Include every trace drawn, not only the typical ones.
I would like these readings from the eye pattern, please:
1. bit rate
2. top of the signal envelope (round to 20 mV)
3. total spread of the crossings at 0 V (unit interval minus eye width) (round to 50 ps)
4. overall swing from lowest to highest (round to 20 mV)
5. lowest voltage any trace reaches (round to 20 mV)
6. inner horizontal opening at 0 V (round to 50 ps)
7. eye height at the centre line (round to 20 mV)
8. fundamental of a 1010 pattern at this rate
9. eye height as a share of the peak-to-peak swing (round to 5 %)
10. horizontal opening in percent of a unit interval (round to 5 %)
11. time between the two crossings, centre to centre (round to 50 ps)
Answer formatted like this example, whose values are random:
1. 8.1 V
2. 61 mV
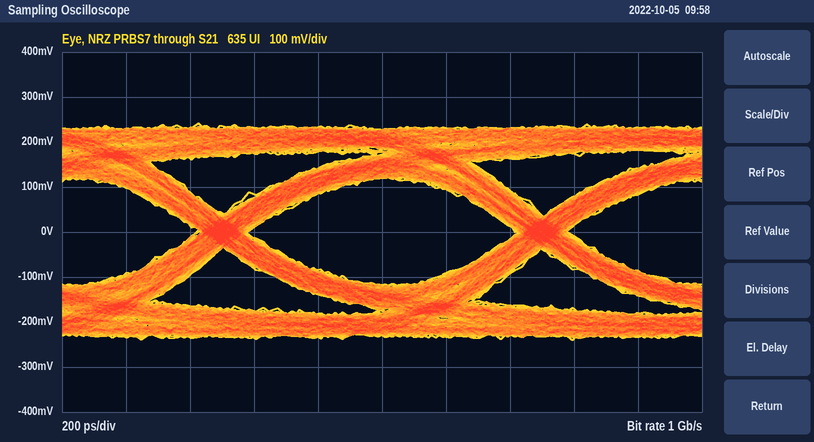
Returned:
1. 1 Gb/s
2. 240 mV
3. 150 ps
4. 480 mV
5. -240 mV
6. 850 ps
7. 240 mV
8. 500 MHz
9. 50 %
10. 85 %
11. 1.00 ns
